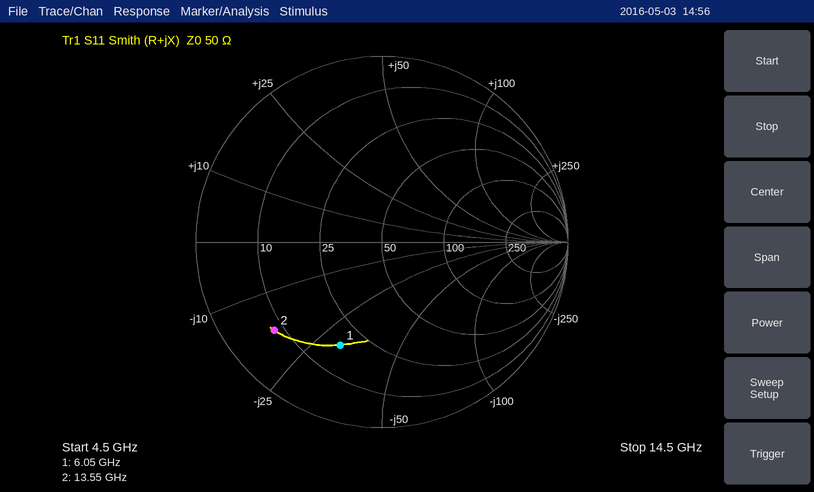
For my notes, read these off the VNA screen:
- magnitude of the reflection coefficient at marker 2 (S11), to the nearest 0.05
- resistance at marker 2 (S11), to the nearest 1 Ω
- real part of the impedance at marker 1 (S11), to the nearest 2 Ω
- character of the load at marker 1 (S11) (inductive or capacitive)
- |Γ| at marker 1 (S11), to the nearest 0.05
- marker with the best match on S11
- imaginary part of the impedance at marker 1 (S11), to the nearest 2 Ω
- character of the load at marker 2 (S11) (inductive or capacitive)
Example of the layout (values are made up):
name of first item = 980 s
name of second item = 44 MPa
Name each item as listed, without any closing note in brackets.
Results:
magnitude of the reflection coefficient at marker 2 (S11), to the nearest 0.05 = 0.75
resistance at marker 2 (S11), to the nearest 1 Ω = 8 Ω
real part of the impedance at marker 1 (S11), to the nearest 2 Ω = 18 Ω
character of the load at marker 1 (S11) = capacitive
|Γ| at marker 1 (S11), to the nearest 0.05 = 0.60
marker with the best match on S11 = marker 1
imaginary part of the impedance at marker 1 (S11), to the nearest 2 Ω = -30 Ω
character of the load at marker 2 (S11) = capacitive
